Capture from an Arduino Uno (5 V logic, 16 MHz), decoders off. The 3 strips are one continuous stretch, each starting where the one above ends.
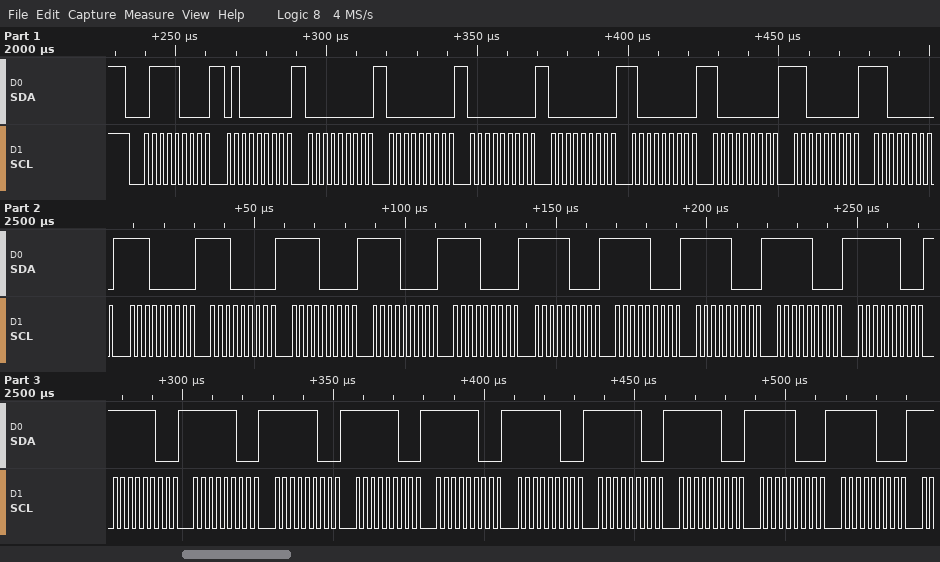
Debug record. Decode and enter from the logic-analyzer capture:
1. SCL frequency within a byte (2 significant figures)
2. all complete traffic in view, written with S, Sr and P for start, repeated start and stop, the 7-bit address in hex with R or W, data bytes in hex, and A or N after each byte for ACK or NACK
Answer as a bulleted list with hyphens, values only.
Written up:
- 400 kHz
- S 3CW A 40 A 00 A 00 A 00 A 00 A 80 A 80 A C0 A C0 A E0 A E0 A F0 A F0 A F0 A F8 A F8 A F8 A F8 A FC A FC A FC A FC A FC A FC A FC A FC A FC A F8 A F8 A
